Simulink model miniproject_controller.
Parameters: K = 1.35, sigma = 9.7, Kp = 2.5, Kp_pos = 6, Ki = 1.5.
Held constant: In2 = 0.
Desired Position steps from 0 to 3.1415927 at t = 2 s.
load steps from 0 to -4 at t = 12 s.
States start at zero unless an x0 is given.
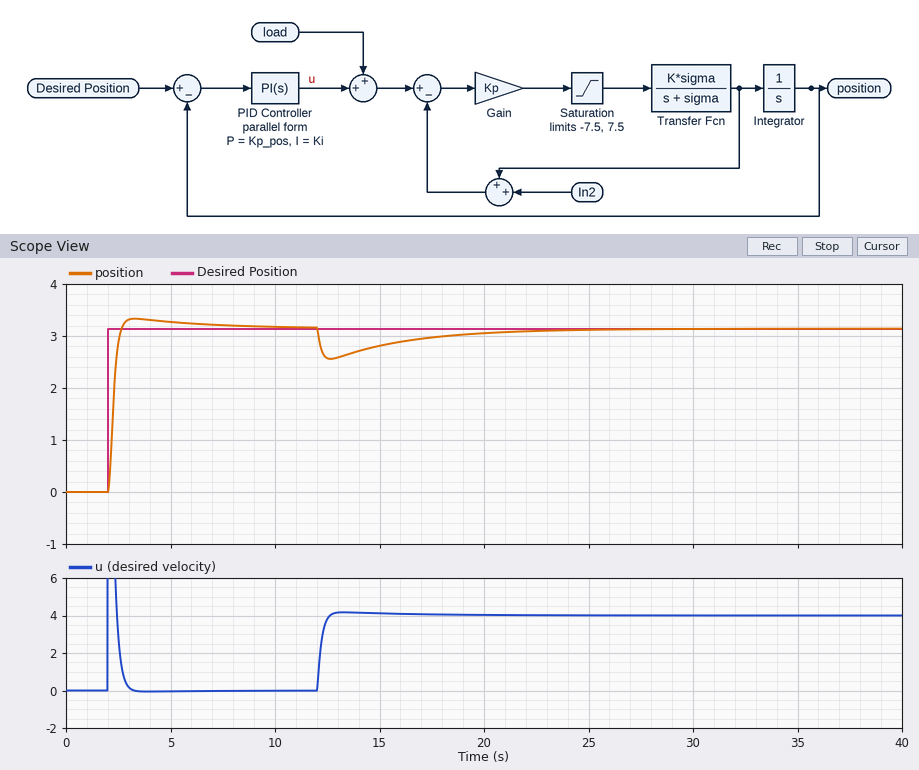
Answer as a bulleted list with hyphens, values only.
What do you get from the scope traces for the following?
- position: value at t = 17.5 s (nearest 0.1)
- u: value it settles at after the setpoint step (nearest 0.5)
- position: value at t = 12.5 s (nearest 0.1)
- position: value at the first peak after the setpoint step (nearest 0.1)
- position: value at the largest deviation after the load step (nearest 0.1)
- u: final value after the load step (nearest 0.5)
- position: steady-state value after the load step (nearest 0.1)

- 3.0
- 0.0
- 2.6
- 3.3
- 2.6
- 4.0
- 3.1
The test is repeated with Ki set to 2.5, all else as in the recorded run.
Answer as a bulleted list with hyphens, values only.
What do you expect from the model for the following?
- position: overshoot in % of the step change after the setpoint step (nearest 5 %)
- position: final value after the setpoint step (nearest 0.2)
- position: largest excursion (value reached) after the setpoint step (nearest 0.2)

- 10 %
- 3.2
- 3.4
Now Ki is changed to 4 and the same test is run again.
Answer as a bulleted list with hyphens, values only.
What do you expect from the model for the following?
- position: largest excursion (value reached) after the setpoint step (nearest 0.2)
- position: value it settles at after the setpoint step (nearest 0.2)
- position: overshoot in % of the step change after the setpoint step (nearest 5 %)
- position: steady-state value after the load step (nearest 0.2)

- 3.6
- 3.2
- 15 %
- 3.2
